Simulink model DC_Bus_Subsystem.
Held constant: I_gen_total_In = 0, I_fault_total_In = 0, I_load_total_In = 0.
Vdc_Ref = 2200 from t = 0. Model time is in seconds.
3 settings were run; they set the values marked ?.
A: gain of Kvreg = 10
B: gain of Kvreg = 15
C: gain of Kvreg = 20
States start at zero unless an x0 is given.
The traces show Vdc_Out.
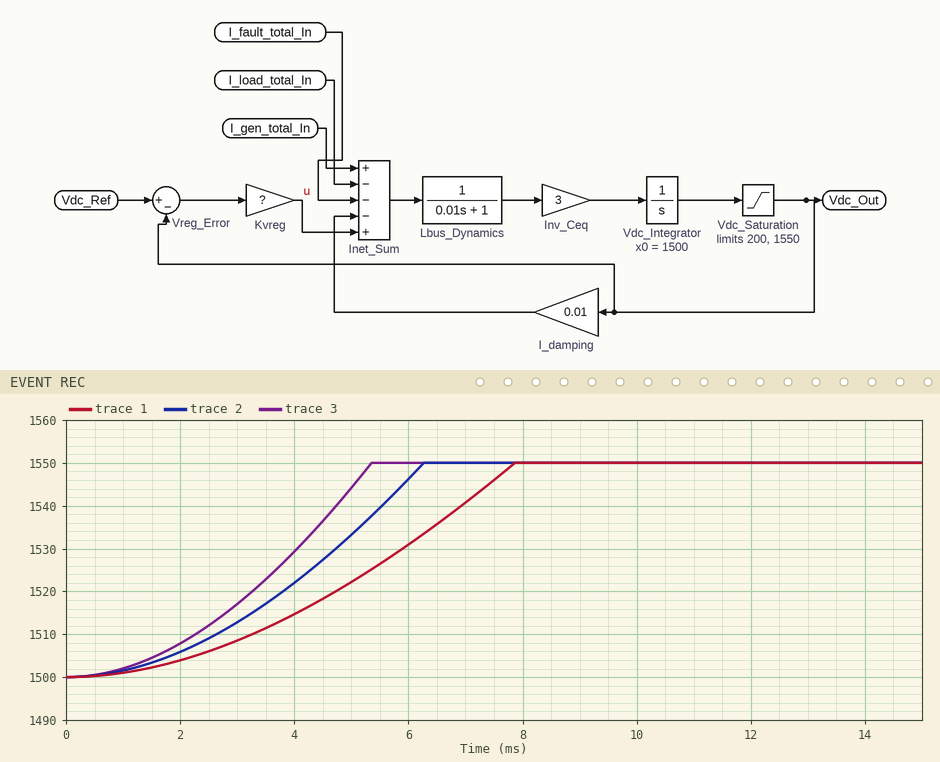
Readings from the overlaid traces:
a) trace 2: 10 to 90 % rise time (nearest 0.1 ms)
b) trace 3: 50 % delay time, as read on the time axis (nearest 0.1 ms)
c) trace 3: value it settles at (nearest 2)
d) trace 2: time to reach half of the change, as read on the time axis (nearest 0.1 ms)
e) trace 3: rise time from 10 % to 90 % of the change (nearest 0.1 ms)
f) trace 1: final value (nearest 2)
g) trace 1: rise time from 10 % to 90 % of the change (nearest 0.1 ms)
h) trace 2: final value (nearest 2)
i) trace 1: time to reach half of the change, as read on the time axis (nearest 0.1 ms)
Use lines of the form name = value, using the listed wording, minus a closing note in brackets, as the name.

trace 2: 10 to 90 % rise time = 4.1 ms
trace 3: 50 % delay time, as read on the time axis = 3.7 ms
trace 3: value it settles at = 1550
trace 2: time to reach half of the change, as read on the time axis = 4.3 ms
trace 3: rise time from 10 % to 90 % of the change = 3.5 ms
trace 1: final value = 1550
trace 1: rise time from 10 % to 90 % of the change = 5.1 ms
trace 2: final value = 1550
trace 1: time to reach half of the change, as read on the time axis = 5.3 ms
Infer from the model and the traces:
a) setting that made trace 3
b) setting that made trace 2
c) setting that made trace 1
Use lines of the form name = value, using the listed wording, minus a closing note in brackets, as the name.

setting that made trace 3 = C
setting that made trace 2 = B
setting that made trace 1 = A
